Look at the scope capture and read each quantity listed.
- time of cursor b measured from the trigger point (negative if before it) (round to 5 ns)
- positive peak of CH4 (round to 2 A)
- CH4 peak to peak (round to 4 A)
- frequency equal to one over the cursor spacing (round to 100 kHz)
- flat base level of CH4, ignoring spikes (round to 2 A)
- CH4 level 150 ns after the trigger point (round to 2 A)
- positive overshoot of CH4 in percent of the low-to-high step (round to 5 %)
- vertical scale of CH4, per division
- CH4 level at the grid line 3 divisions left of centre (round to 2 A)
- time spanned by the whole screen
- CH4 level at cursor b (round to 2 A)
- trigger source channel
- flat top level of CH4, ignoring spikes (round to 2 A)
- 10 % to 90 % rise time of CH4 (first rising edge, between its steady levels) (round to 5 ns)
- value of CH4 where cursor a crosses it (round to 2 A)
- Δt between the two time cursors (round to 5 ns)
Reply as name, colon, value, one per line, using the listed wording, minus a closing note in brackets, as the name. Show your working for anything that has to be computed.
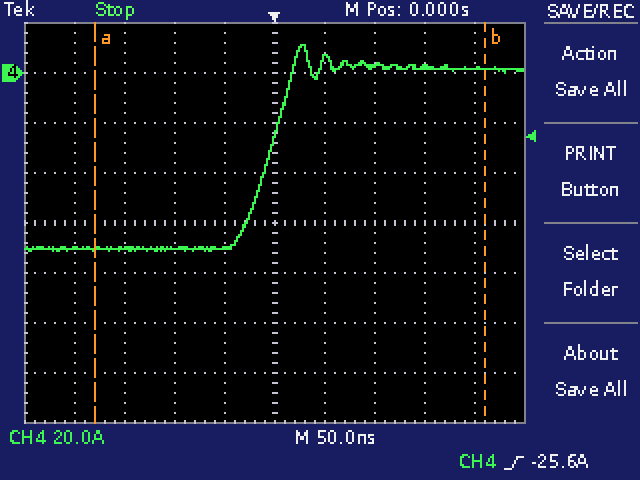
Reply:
time of cursor b measured from the trigger point (negative if before it): +210 ns
positive peak of CH4: 12 A
CH4 peak to peak: 84 A
frequency equal to one over the cursor spacing: 1 / 390 ns ≈ 2.6 MHz
flat base level of CH4, ignoring spikes: -70 A
CH4 level 150 ns after the trigger point: 2 A
positive overshoot of CH4 in percent of the low-to-high step: 15 %
vertical scale of CH4, per division: 20 A
CH4 level at the grid line 3 divisions left of centre: -70 A
time spanned by the whole screen: 500 ns
CH4 level at cursor b: 2 A
trigger source channel: CH4
flat top level of CH4, ignoring spikes: 2 A
10 % to 90 % rise time of CH4 (first rising edge, between its steady levels): 45 ns
value of CH4 where cursor a crosses it: -70 A
Δt between the two time cursors: 390 ns
